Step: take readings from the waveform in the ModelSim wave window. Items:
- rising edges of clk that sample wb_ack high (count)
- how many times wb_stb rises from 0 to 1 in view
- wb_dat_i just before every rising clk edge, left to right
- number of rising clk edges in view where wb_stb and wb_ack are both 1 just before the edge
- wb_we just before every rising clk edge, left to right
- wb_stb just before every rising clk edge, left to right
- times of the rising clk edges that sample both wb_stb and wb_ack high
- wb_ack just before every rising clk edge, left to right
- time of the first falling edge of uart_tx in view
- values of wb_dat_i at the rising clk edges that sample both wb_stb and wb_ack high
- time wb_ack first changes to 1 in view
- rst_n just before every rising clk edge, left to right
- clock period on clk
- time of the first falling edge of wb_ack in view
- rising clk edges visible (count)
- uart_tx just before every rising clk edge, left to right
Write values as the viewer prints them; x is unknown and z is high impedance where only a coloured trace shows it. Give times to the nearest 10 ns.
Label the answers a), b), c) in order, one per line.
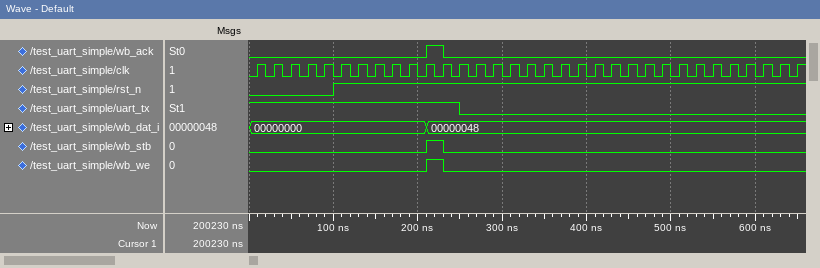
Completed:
a) 1
b) 1
c) 00000000, 00000000, 00000000, 00000000, 00000000, 00000000, 00000000, 00000000, 00000000, 00000000, 00000000, 00000048, 00000048, 00000048, 00000048, 00000048, 00000048, 00000048, 00000048, 00000048, 00000048, 00000048, 00000048, 00000048, 00000048, 00000048, 00000048, 00000048, 00000048, 00000048, 00000048, 00000048, 00000048
d) 1
e) 0 0 0 0 0 0 0 0 0 0 0 1 0 0 0 0 0 0 0 0 0 0 0 0 0 0 0 0 0 0 0 0 0
f) 0 0 0 0 0 0 0 0 0 0 0 1 0 0 0 0 0 0 0 0 0 0 0 0 0 0 0 0 0 0 0 0 0
g) 230 ns
h) 0 0 0 0 0 0 0 0 0 0 0 1 0 0 0 0 0 0 0 0 0 0 0 0 0 0 0 0 0 0 0 0 0
i) 250 ns
j) 00000048
k) 210 ns
l) 0 0 0 0 0 1 1 1 1 1 1 1 1 1 1 1 1 1 1 1 1 1 1 1 1 1 1 1 1 1 1 1 1
m) 20 ns
n) 230 ns
o) 33
p) 1 1 1 1 1 1 1 1 1 1 1 1 1 0 0 0 0 0 0 0 0 0 0 0 0 0 0 0 0 0 0 0 0
